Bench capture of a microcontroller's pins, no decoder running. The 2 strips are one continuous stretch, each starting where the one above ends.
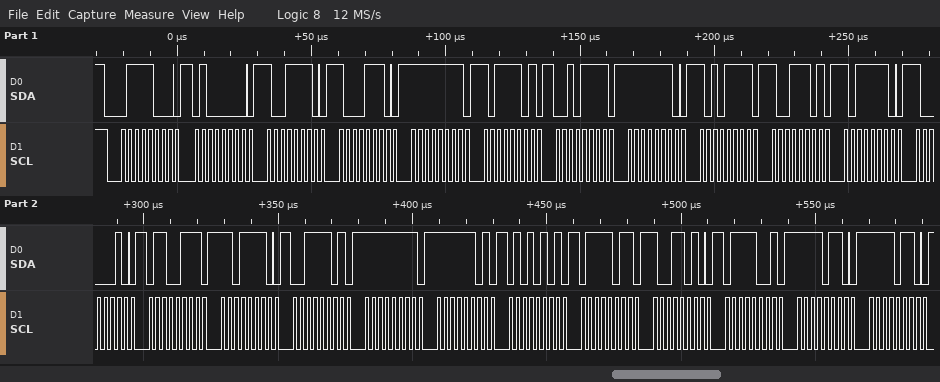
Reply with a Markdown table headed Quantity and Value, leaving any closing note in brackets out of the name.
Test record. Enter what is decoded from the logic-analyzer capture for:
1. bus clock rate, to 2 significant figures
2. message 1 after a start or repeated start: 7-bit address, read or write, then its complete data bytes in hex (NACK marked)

| Quantity | Value |
|---|---|
| bus clock rate, to 2 significant figures | 400 kHz |
| message 1 after a start or repeated start: 7-bit address, read or write, then its complete data bytes in hex | 0x3C write: 40 9E 8E FF BD 2F FE AF 9D BE 82 67 DE 3D FF FD 55 7B 9A 79 F6 F6 |
